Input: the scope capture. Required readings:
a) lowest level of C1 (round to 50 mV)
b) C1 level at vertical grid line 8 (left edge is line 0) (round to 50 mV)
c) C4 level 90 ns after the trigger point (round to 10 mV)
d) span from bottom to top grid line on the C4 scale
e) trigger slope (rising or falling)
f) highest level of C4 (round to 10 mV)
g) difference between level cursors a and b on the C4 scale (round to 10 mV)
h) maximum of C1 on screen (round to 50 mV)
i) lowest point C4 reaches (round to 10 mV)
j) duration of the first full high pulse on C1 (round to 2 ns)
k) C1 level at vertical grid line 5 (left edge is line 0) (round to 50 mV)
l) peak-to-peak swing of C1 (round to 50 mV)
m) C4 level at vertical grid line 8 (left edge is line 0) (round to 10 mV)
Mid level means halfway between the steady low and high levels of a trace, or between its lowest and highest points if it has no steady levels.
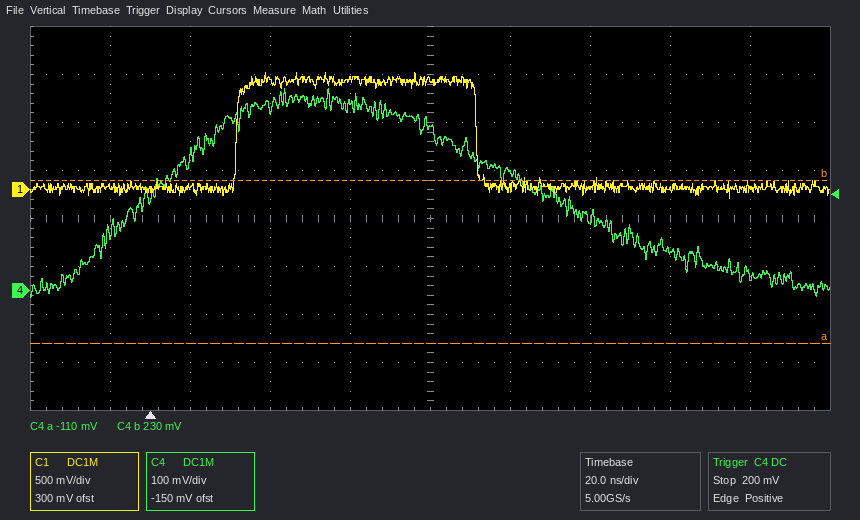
-100 mV
0 mV
250 mV
800 mV
rising
420 mV
340 mV
1.20 V
-10 mV
60 ns
1.15 V
1.30 V
80 mV
